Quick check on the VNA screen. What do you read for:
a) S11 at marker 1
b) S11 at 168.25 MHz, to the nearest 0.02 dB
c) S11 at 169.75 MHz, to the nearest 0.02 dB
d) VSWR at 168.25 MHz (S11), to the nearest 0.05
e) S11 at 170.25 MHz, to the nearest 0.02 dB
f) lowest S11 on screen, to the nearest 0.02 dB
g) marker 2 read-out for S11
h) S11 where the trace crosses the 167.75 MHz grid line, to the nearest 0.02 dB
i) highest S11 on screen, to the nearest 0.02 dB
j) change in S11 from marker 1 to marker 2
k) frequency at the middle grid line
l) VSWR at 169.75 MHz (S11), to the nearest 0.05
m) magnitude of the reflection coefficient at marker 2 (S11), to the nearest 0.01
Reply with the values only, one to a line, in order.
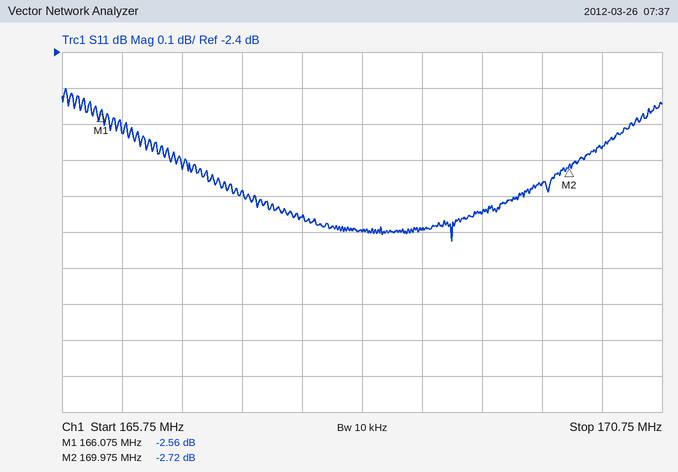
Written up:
-2.56 dB
-2.90 dB
-2.76 dB
6.05
-2.66 dB
-2.92 dB
-2.72 dB
-2.86 dB
-2.50 dB
-0.16 dB
168.25 MHz
6.35
0.73
